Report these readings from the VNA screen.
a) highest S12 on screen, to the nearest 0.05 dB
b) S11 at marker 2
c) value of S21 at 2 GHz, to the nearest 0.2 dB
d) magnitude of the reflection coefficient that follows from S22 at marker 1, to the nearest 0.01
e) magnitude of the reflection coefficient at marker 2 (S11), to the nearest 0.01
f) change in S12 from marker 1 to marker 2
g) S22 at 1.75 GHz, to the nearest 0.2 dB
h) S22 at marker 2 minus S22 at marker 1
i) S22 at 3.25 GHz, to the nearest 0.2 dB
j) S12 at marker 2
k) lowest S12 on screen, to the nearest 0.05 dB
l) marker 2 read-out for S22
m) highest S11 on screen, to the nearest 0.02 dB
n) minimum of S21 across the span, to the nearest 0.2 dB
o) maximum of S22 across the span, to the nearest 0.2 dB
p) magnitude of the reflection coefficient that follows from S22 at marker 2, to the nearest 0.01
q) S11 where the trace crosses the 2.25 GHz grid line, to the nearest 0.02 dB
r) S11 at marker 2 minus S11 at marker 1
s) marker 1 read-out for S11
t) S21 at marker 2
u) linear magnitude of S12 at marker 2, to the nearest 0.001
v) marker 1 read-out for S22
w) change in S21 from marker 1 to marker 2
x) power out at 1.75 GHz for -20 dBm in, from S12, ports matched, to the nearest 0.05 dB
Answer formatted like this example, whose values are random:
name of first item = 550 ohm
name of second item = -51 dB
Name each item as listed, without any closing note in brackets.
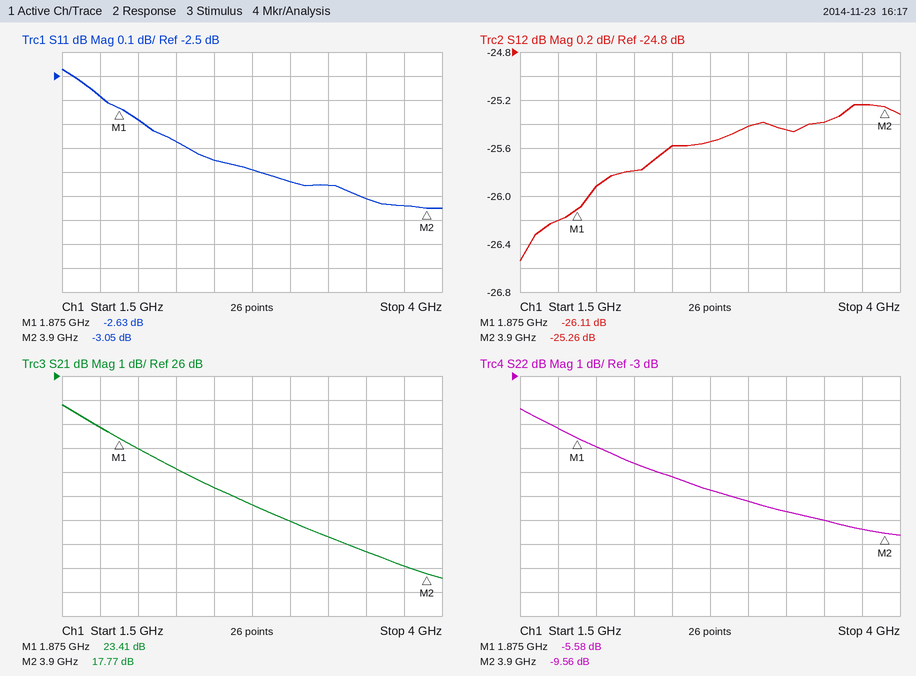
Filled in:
highest S12 on screen, to the nearest 0.05 dB = -25.25 dB
S11 at marker 2 = -3.05 dB
value of S21 at 2 GHz, to the nearest 0.2 dB = 23.0 dB
magnitude of the reflection coefficient that follows from S22 at marker 1, to the nearest 0.01 = 0.53
magnitude of the reflection coefficient at marker 2 (S11), to the nearest 0.01 = 0.70
change in S12 from marker 1 to marker 2 = 0.85 dB
S22 at 1.75 GHz, to the nearest 0.2 dB = -5.2 dB
S22 at marker 2 minus S22 at marker 1 = -3.98 dB
S22 at 3.25 GHz, to the nearest 0.2 dB = -8.6 dB
S12 at marker 2 = -25.26 dB
lowest S12 on screen, to the nearest 0.05 dB = -26.55 dB
marker 2 read-out for S22 = -9.56 dB
highest S11 on screen, to the nearest 0.02 dB = -2.48 dB
minimum of S21 across the span, to the nearest 0.2 dB = 17.6 dB
maximum of S22 across the span, to the nearest 0.2 dB = -4.4 dB
magnitude of the reflection coefficient that follows from S22 at marker 2, to the nearest 0.01 = 0.33
S11 where the trace crosses the 2.25 GHz grid line, to the nearest 0.02 dB = -2.78 dB
S11 at marker 2 minus S11 at marker 1 = -0.42 dB
marker 1 read-out for S11 = -2.63 dB
S21 at marker 2 = 17.77 dB
linear magnitude of S12 at marker 2, to the nearest 0.001 = 0.055
marker 1 read-out for S22 = -5.58 dB
change in S21 from marker 1 to marker 2 = -5.64 dB
power out at 1.75 GHz for -20 dBm in, from S12, ports matched, to the nearest 0.05 dB = -46.20 dBm
